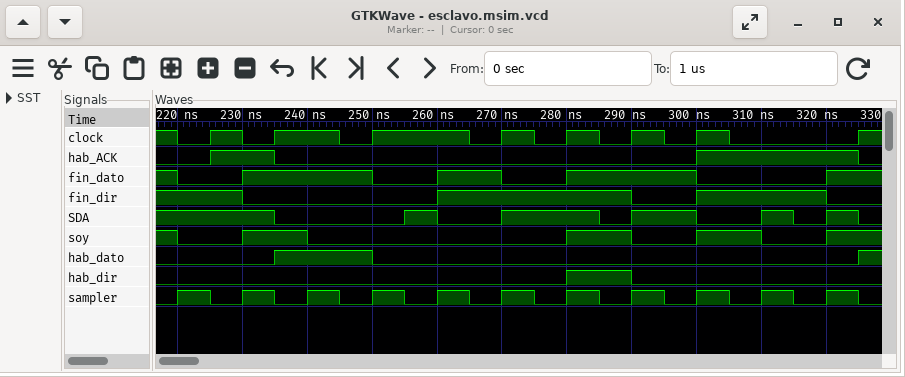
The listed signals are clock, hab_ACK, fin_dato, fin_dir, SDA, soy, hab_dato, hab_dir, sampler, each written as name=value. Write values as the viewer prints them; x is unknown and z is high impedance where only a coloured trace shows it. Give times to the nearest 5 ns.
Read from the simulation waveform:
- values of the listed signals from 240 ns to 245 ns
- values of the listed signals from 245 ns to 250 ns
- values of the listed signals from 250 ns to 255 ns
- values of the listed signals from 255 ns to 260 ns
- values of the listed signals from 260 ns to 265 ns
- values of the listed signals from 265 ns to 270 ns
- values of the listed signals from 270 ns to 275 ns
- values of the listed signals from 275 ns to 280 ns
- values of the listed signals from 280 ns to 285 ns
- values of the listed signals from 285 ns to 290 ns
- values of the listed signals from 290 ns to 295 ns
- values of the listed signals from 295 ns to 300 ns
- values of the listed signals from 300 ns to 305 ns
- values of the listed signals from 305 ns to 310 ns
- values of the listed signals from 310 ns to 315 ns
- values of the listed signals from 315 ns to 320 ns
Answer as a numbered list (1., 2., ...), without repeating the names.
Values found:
1. clock=1, hab_ACK=0, fin_dato=1, fin_dir=0, SDA=0, soy=0, hab_dato=1, hab_dir=0, sampler=1
2. clock=0, hab_ACK=0, fin_dato=1, fin_dir=0, SDA=0, soy=0, hab_dato=1, hab_dir=0, sampler=0
3. clock=1, hab_ACK=0, fin_dato=0, fin_dir=0, SDA=0, soy=0, hab_dato=0, hab_dir=0, sampler=1
4. clock=1, hab_ACK=0, fin_dato=0, fin_dir=0, SDA=1, soy=0, hab_dato=0, hab_dir=0, sampler=0
5. clock=1, hab_ACK=0, fin_dato=1, fin_dir=1, SDA=0, soy=0, hab_dato=0, hab_dir=0, sampler=1
6. clock=0, hab_ACK=0, fin_dato=1, fin_dir=1, SDA=0, soy=0, hab_dato=0, hab_dir=0, sampler=0
7. clock=1, hab_ACK=0, fin_dato=0, fin_dir=1, SDA=1, soy=0, hab_dato=0, hab_dir=0, sampler=1
8. clock=0, hab_ACK=0, fin_dato=0, fin_dir=1, SDA=1, soy=0, hab_dato=0, hab_dir=0, sampler=0
9. clock=1, hab_ACK=0, fin_dato=1, fin_dir=1, SDA=1, soy=1, hab_dato=0, hab_dir=1, sampler=1
10. clock=0, hab_ACK=0, fin_dato=1, fin_dir=1, SDA=0, soy=1, hab_dato=0, hab_dir=1, sampler=0
11. clock=1, hab_ACK=0, fin_dato=1, fin_dir=0, SDA=1, soy=0, hab_dato=0, hab_dir=0, sampler=1
12. clock=0, hab_ACK=0, fin_dato=1, fin_dir=0, SDA=1, soy=0, hab_dato=0, hab_dir=0, sampler=0
13. clock=1, hab_ACK=1, fin_dato=0, fin_dir=1, SDA=0, soy=1, hab_dato=0, hab_dir=0, sampler=1
14. clock=0, hab_ACK=1, fin_dato=0, fin_dir=1, SDA=0, soy=1, hab_dato=0, hab_dir=0, sampler=0
15. clock=0, hab_ACK=1, fin_dato=0, fin_dir=1, SDA=1, soy=0, hab_dato=0, hab_dir=0, sampler=1
16. clock=0, hab_ACK=1, fin_dato=0, fin_dir=1, SDA=0, soy=0, hab_dato=0, hab_dir=0, sampler=0
